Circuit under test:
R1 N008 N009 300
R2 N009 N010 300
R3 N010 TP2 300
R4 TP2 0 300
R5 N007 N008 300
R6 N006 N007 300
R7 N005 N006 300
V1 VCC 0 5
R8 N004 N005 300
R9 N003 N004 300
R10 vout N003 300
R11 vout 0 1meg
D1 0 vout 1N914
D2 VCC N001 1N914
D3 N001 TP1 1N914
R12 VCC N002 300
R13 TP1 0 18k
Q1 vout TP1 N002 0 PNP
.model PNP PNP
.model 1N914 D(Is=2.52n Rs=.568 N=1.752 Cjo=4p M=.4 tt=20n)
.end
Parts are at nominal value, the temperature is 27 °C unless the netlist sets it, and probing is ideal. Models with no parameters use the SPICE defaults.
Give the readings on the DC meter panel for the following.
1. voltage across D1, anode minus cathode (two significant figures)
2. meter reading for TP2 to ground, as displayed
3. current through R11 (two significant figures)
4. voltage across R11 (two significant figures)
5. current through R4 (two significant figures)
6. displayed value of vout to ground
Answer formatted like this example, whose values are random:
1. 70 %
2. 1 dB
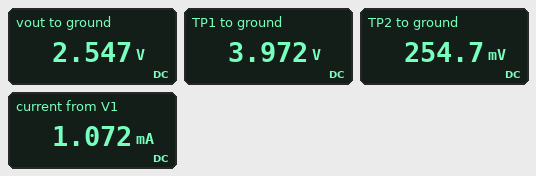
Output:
1. -2.5 V
2. 254.7 mV
3. 2.5 µA
4. 2.5 V
5. 850 µA
6. 2.547 V
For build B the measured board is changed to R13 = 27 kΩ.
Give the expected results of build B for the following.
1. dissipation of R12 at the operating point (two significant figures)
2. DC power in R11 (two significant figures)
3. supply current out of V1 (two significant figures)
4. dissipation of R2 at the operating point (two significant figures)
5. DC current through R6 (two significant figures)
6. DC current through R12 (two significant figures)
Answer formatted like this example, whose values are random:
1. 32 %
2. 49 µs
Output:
1. 170 µW
2. 4.9 µW
3. 890 µA
4. 160 µW
5. 740 µA
6. 750 µA
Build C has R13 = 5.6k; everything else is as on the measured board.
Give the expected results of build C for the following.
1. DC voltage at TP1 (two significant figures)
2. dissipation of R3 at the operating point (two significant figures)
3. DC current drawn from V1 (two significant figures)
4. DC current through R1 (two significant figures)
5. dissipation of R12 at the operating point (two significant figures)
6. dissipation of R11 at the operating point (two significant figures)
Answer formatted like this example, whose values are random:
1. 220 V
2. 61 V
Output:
1. 3.9 V
2. 410 µW
3. 1.9 mA
4. 1.2 mA
5. 420 µW
6. 12 µW
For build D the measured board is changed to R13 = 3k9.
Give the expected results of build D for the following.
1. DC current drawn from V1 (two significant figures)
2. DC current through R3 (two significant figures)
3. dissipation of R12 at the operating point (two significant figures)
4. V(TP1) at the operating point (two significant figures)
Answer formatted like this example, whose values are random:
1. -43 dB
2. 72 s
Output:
1. 2.3 mA
2. 1.3 mA
3. 500 µW
4. 3.8 V
